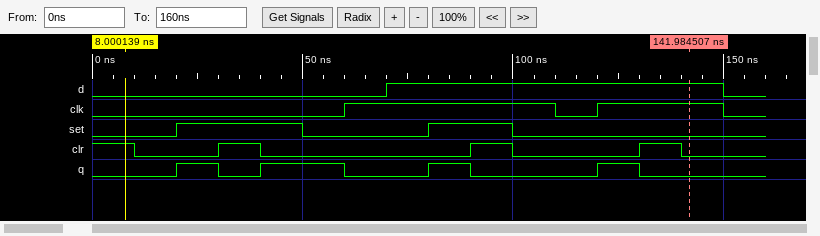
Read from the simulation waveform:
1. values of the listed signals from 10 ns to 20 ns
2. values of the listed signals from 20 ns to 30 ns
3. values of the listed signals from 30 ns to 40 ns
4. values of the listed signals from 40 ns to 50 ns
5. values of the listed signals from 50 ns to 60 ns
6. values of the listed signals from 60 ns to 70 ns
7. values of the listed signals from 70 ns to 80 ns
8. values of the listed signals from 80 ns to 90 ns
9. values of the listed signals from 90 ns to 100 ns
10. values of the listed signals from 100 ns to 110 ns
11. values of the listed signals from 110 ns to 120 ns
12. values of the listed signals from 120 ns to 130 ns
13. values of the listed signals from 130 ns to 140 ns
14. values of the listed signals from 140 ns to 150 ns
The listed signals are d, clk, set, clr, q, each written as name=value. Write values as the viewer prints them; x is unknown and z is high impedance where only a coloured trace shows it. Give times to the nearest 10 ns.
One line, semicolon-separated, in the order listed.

d=0, clk=0, set=0, clr=0, q=0; d=0, clk=0, set=1, clr=0, q=1; d=0, clk=0, set=1, clr=1, q=0; d=0, clk=0, set=1, clr=0, q=1; d=0, clk=0, set=0, clr=0, q=1; d=0, clk=1, set=0, clr=0, q=0; d=1, clk=1, set=0, clr=0, q=0; d=1, clk=1, set=1, clr=0, q=1; d=1, clk=1, set=1, clr=1, q=0; d=1, clk=1, set=0, clr=0, q=0; d=1, clk=0, set=0, clr=0, q=0; d=1, clk=1, set=0, clr=0, q=1; d=1, clk=1, set=0, clr=1, q=0; d=1, clk=1, set=0, clr=0, q=0
